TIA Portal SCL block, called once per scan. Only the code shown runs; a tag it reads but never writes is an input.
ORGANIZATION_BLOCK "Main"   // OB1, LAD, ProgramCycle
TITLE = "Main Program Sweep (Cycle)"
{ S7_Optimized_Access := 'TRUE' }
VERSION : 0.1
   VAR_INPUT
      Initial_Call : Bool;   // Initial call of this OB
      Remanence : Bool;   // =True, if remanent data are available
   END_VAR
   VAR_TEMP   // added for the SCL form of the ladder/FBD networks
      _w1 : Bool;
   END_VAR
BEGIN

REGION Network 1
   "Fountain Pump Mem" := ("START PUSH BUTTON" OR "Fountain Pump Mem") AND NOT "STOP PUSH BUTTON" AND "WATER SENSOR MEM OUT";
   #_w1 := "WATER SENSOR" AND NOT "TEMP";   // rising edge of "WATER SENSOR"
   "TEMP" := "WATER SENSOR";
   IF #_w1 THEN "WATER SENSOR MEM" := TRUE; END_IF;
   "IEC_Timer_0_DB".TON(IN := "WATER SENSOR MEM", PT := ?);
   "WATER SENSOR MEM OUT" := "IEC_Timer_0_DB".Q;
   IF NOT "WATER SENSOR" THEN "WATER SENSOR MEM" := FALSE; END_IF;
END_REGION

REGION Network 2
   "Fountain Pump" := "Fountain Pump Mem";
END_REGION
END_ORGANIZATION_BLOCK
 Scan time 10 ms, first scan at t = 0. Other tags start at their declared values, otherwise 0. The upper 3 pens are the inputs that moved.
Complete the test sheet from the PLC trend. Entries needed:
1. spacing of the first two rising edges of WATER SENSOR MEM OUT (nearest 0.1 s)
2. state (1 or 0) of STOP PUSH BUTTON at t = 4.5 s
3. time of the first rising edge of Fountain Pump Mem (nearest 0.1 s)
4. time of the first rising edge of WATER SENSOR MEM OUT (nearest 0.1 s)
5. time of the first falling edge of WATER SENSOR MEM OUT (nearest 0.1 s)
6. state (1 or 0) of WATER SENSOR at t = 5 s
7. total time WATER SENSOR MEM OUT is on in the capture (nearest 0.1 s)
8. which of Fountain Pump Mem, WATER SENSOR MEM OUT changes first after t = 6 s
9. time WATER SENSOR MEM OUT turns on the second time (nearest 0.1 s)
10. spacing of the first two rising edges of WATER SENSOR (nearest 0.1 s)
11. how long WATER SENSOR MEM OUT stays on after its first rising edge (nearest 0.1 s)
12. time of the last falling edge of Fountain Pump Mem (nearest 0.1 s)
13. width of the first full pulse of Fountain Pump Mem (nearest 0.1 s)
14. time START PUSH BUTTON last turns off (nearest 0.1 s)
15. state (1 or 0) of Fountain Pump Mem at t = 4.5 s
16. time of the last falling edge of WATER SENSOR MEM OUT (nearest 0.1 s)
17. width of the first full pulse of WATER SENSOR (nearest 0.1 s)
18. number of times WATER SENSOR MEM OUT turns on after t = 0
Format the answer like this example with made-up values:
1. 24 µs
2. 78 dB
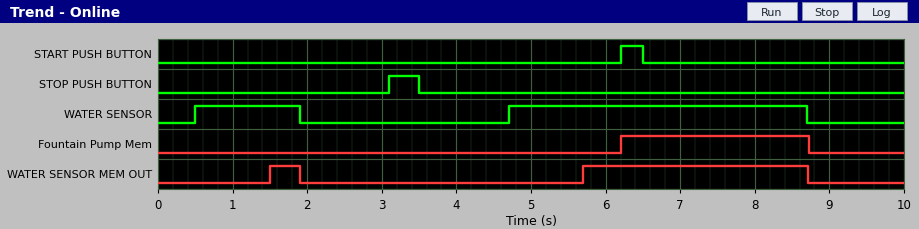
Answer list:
1. 4.2 s
2. 0
3. 6.2 s
4. 1.5 s
5. 1.9 s
6. 1
7. 3.4 s
8. Fountain Pump Mem
9. 5.7 s
10. 4.2 s
11. 0.4 s
12. 8.7 s
13. 2.5 s
14. 6.5 s
15. 0
16. 8.7 s
17. 1.4 s
18. 2
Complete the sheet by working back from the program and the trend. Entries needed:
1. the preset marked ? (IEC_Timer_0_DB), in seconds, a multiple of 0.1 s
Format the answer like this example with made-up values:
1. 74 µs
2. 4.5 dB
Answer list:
1. 1.0 s
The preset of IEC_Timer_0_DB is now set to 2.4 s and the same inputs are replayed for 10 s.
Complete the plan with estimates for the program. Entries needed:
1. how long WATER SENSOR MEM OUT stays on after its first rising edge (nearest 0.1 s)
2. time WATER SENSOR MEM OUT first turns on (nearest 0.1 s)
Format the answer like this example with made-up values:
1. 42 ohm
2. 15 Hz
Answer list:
1. 1.6 s
2. 7.1 s
